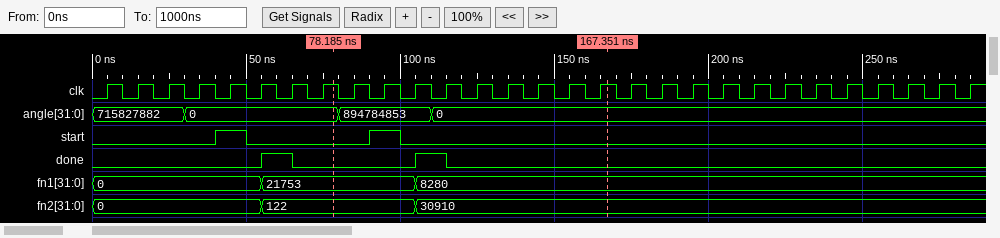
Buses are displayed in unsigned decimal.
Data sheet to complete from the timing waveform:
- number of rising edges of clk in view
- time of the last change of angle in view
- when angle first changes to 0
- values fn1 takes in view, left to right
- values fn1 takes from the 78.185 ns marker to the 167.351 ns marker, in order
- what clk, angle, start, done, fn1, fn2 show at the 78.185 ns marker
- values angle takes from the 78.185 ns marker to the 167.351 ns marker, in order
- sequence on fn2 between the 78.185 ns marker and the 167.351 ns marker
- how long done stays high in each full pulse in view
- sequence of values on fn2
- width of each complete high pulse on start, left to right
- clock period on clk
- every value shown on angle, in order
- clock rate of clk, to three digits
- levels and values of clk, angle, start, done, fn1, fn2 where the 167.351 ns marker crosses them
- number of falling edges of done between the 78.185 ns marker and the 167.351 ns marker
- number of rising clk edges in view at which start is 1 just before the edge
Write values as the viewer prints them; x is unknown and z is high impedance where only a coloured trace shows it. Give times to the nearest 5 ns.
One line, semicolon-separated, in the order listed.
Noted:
29; 110 ns; 30 ns; 0, 21753, 8280; 21753, 8280; clk=1, angle=0, start=0, done=0, fn1=21753, fn2=122; 0, 894784853, 0; 122, 30910; 10 ns, 10 ns; 0, 122, 30910; 10 ns, 10 ns; 10 ns; 715827882, 0, 894784853, 0; 100 MHz; clk=1, angle=0, start=0, done=0, fn1=8280, fn2=30910; 1; 2
